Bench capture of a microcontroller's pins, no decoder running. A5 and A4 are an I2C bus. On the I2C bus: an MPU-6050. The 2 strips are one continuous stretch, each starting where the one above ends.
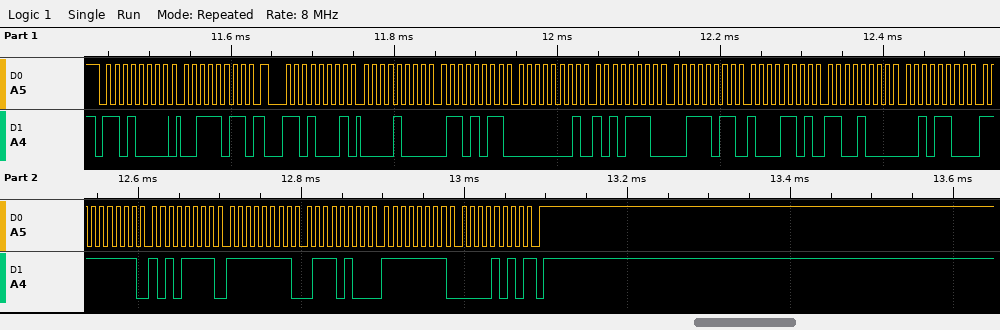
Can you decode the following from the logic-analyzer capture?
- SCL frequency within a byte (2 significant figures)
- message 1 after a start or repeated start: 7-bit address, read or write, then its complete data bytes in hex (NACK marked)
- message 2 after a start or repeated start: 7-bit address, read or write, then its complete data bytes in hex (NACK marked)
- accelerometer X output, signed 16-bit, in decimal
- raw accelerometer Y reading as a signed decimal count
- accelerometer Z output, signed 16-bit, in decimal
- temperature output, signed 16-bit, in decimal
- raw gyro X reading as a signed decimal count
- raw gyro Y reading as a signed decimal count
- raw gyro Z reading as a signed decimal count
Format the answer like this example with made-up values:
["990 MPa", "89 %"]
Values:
["100 kHz", "0x68 write: 3B", "0x68 read: 08 6B 01 AE 3B 8D C8 2C FF AF FF 74 FF 0A NACK", "2155", "430", "15245", "-14292", "-81", "-140", "-246"]
